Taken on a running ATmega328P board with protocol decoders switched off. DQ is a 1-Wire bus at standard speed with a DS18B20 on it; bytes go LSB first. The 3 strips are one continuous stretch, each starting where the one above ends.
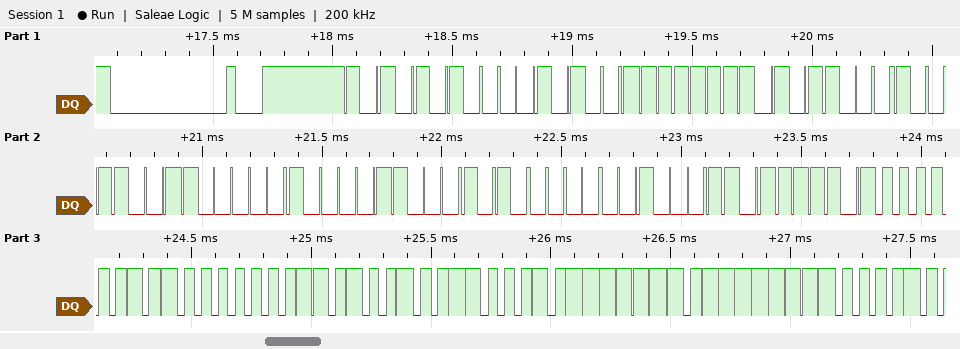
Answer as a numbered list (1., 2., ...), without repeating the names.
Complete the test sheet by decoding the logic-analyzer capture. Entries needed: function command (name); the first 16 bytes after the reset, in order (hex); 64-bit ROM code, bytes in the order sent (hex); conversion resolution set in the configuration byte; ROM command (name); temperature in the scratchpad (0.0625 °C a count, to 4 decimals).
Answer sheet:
1. Read Scratchpad
2. 55 28 FF 1A 99 41 18 05 C4 BE 40 01 4B 46 7F FF
3. 28 FF 1A 99 41 18 05 C4
4. 12 bits
5. Match ROM
6. 20.0000 °C
